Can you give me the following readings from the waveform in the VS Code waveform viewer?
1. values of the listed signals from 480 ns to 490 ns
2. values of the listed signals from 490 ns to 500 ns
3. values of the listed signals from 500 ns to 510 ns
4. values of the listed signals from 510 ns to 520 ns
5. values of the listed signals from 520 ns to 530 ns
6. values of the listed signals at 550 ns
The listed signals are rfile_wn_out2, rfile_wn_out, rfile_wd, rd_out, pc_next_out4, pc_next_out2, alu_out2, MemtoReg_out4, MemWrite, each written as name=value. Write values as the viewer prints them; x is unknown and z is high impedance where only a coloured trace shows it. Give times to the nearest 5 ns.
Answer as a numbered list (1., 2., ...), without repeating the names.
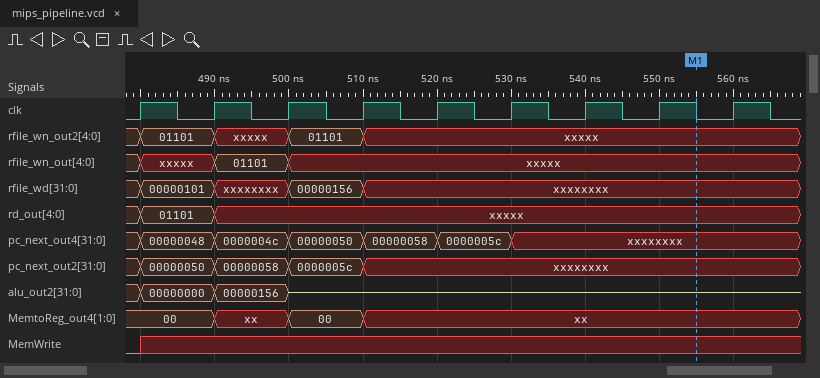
1. rfile_wn_out2=01101, rfile_wn_out=xxxxx, rfile_wd=00000101, rd_out=01101, pc_next_out4=00000048, pc_next_out2=00000050, alu_out2=00000000, MemtoReg_out4=00, MemWrite=x
2. rfile_wn_out2=xxxxx, rfile_wn_out=01101, rfile_wd=xxxxxxxx, rd_out=xxxxx, pc_next_out4=0000004c, pc_next_out2=00000058, alu_out2=00000156, MemtoReg_out4=xx, MemWrite=x
3. rfile_wn_out2=01101, rfile_wn_out=xxxxx, rfile_wd=00000156, rd_out=xxxxx, pc_next_out4=00000050, pc_next_out2=0000005c, alu_out2=z, MemtoReg_out4=00, MemWrite=x
4. rfile_wn_out2=xxxxx, rfile_wn_out=xxxxx, rfile_wd=xxxxxxxx, rd_out=xxxxx, pc_next_out4=00000058, pc_next_out2=xxxxxxxx, alu_out2=z, MemtoReg_out4=xx, MemWrite=x
5. rfile_wn_out2=xxxxx, rfile_wn_out=xxxxx, rfile_wd=xxxxxxxx, rd_out=xxxxx, pc_next_out4=0000005c, pc_next_out2=xxxxxxxx, alu_out2=z, MemtoReg_out4=xx, MemWrite=x
6. rfile_wn_out2=xxxxx, rfile_wn_out=xxxxx, rfile_wd=xxxxxxxx, rd_out=xxxxx, pc_next_out4=xxxxxxxx, pc_next_out2=xxxxxxxx, alu_out2=z, MemtoReg_out4=xx, MemWrite=x
